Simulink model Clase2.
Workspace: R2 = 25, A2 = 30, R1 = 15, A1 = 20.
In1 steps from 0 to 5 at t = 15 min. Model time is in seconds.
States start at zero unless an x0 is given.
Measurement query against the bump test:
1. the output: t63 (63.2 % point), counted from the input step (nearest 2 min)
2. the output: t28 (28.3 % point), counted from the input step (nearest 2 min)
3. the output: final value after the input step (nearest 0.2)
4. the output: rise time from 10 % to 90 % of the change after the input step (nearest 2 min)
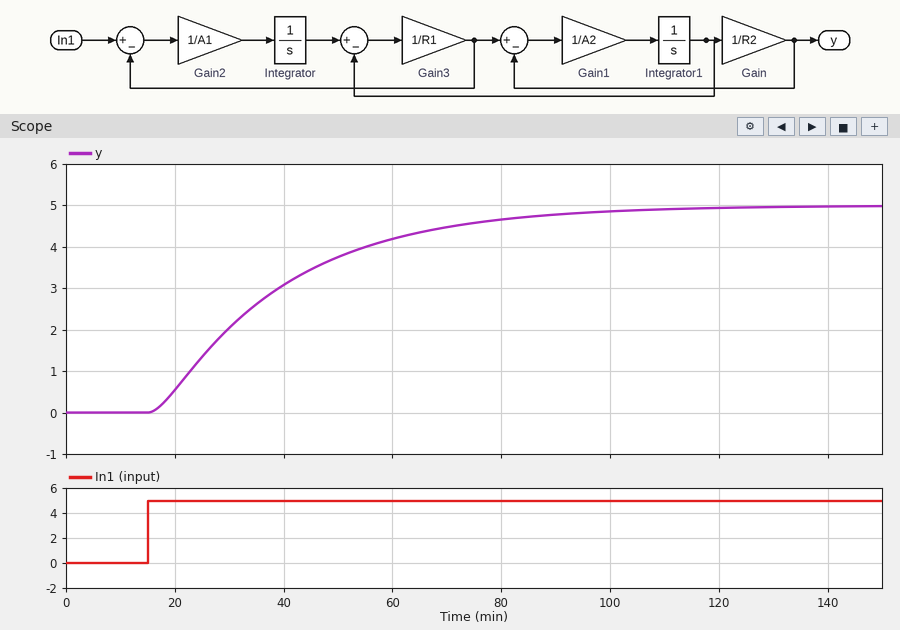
26 min
10 min
5.0
52 min
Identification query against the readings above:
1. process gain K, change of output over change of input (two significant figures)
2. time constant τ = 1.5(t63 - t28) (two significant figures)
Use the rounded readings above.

1.0
24 min
